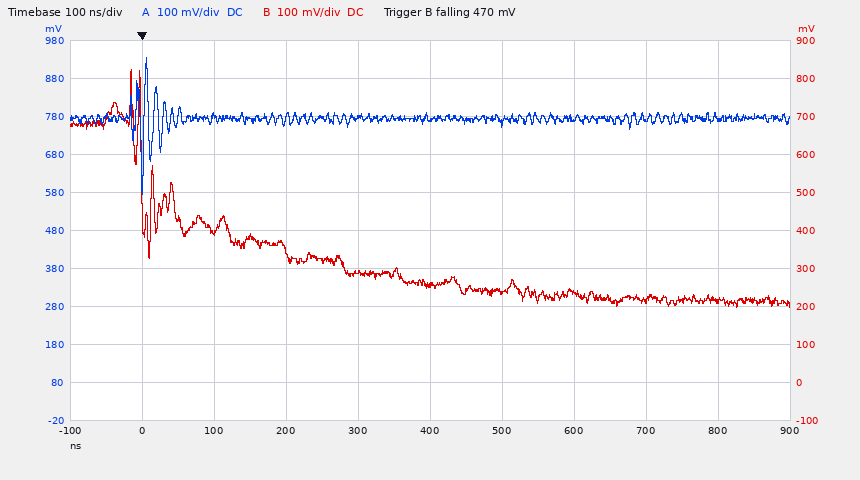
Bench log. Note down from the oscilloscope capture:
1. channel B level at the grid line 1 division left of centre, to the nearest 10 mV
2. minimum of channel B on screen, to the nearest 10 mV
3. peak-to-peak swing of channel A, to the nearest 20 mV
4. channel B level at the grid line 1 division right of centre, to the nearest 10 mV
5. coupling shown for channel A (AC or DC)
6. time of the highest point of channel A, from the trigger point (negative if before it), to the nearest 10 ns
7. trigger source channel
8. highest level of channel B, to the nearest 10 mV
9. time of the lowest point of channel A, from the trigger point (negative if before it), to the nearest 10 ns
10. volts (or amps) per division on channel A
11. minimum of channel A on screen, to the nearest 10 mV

290 mV
200 mV
360 mV
240 mV
DC
+10 ns
channel B
820 mV
0 ns
100 mV
570 mV
